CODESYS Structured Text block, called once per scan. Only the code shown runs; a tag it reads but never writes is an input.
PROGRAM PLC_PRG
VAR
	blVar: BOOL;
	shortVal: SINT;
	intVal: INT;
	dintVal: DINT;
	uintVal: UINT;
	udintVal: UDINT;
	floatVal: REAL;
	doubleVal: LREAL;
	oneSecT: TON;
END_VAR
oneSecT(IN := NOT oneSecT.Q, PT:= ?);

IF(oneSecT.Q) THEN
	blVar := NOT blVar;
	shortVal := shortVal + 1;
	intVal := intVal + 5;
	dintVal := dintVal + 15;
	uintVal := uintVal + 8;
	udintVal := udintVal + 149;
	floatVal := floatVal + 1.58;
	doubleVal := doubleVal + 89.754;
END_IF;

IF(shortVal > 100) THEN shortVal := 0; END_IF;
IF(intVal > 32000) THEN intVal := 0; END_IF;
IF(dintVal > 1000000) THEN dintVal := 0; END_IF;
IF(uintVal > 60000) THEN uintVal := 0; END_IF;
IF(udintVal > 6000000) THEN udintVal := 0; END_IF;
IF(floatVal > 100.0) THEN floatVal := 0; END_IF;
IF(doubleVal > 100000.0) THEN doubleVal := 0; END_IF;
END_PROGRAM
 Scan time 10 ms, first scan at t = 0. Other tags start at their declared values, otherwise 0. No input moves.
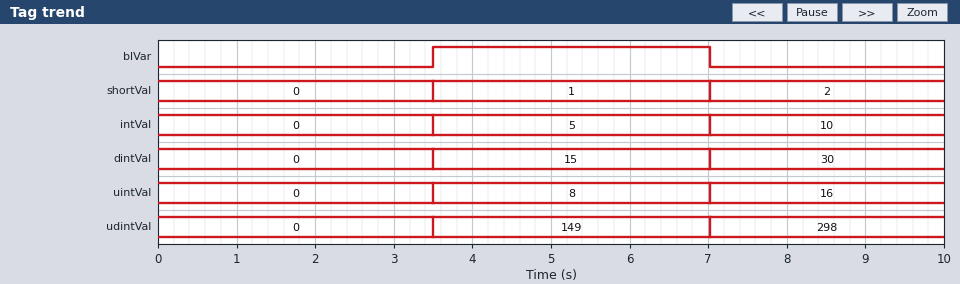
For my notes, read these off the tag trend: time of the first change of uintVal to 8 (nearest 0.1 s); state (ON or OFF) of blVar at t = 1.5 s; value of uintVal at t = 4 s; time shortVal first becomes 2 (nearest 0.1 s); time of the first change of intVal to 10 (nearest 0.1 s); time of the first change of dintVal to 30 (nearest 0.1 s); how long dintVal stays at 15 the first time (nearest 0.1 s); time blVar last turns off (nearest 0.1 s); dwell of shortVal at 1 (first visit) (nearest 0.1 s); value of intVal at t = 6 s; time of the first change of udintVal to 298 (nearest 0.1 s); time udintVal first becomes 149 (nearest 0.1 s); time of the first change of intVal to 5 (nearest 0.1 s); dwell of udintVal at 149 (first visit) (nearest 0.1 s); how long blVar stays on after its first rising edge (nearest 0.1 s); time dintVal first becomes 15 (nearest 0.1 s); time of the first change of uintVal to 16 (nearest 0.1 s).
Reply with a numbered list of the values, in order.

1. 3.5 s
2. OFF
3. 8
4. 7.0 s
5. 7.0 s
6. 7.0 s
7. 3.5 s
8. 7.0 s
9. 3.5 s
10. 5
11. 7.0 s
12. 3.5 s
13. 3.5 s
14. 3.5 s
15. 3.5 s
16. 3.5 s
17. 7.0 s
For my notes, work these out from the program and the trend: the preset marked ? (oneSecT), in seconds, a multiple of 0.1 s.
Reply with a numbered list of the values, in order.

1. 3.5 s
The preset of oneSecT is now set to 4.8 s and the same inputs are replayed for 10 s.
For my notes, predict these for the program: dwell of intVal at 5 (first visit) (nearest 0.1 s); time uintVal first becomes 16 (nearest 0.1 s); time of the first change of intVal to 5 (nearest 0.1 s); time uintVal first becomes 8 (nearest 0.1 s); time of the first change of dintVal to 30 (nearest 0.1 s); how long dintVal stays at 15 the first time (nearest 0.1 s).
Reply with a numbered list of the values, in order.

1. 4.8 s
2. 9.6 s
3. 4.8 s
4. 4.8 s
5. 9.6 s
6. 4.8 s
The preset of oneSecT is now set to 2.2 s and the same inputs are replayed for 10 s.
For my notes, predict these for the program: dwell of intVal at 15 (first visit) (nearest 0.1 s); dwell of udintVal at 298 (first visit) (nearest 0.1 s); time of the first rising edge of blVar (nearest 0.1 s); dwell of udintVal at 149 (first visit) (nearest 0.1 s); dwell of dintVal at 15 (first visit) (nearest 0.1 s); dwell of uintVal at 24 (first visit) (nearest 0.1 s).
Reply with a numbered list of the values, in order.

1. 2.2 s
2. 2.2 s
3. 2.2 s
4. 2.2 s
5. 2.2 s
6. 2.2 s
